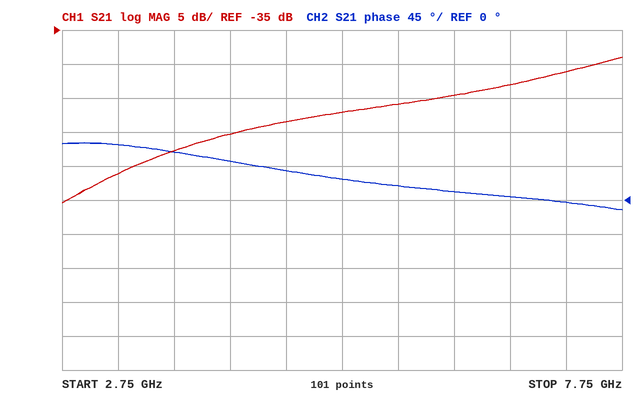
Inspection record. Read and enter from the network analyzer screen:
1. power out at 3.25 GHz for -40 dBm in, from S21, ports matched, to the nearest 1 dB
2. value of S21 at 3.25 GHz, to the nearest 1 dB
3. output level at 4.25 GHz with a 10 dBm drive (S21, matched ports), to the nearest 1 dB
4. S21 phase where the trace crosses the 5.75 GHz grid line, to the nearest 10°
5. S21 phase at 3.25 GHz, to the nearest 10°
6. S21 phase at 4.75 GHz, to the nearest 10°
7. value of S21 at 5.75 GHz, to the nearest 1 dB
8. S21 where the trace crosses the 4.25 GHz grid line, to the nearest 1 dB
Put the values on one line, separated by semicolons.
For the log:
-96 dBm; -56 dB; -40 dBm; 20°; 70°; 40°; -46 dB; -50 dB
